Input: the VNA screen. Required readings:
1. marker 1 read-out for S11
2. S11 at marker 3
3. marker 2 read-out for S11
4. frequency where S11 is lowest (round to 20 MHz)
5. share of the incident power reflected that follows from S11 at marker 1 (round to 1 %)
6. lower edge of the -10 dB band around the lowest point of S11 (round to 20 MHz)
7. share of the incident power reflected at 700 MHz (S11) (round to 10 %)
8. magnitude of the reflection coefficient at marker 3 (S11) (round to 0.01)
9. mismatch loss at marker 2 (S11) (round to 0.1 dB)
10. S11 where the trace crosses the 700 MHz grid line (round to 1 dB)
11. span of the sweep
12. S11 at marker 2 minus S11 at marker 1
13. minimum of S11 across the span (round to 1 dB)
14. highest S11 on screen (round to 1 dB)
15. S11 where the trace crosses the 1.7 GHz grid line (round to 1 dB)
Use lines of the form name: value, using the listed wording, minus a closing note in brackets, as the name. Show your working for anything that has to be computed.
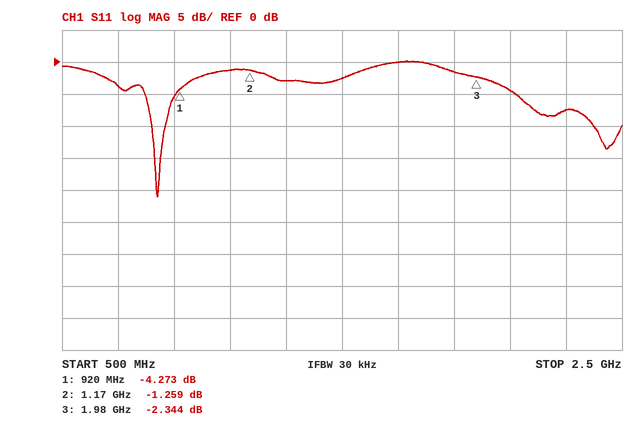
marker 1 read-out for S11: -4.273 dB
S11 at marker 3: -2.344 dB
marker 2 read-out for S11: -1.259 dB
frequency where S11 is lowest: 840 MHz
share of the incident power reflected that follows from S11 at marker 1: 10^(-4.273/10) ≈ 37 %
lower edge of the -10 dB band around the lowest point of S11: 820 MHz
share of the incident power reflected at 700 MHz (S11): 10^(-4/10) ≈ 40 %
magnitude of the reflection coefficient at marker 3 (S11): 10^(-2.344/20) ≈ 0.76
mismatch loss at marker 2 (S11): −10 log10(1 − 10^(-1.259/10)) ≈ 6.0 dB
S11 where the trace crosses the 700 MHz grid line: -4 dB
span of the sweep: 2 GHz
S11 at marker 2 minus S11 at marker 1: -1.259 − (-4.273) = 3.014 dB
minimum of S11 across the span: -21 dB
highest S11 on screen: 0 dB
S11 where the trace crosses the 1.7 GHz grid line: 0 dB
